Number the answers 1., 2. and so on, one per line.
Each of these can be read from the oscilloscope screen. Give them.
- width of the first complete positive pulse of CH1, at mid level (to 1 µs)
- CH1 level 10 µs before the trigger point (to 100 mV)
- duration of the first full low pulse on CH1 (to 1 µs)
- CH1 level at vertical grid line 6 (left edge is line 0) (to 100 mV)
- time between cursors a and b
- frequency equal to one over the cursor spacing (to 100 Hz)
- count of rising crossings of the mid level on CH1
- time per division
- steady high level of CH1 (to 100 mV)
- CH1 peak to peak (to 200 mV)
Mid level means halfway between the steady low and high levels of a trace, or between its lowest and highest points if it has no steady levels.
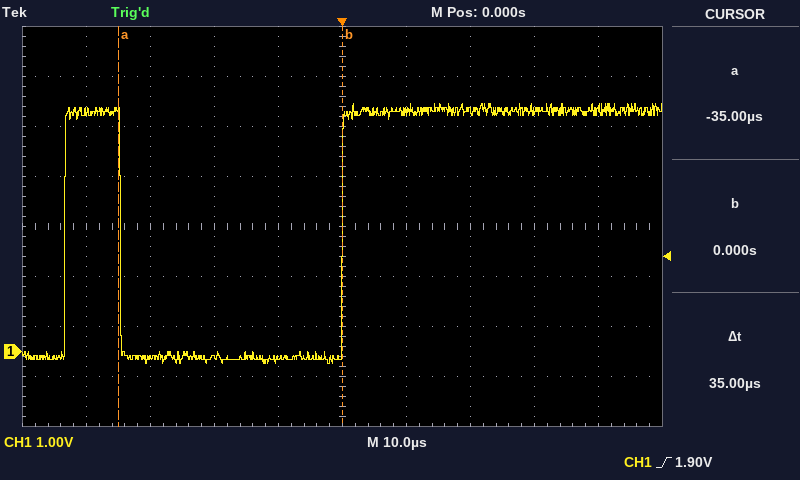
1. 9 µs
2. -200 mV
3. 35 µs
4. 4.8 V
5. 35 µs
6. 28.6 kHz
7. 2
8. 10 µs
9. 4.8 V
10. 5.2 V
